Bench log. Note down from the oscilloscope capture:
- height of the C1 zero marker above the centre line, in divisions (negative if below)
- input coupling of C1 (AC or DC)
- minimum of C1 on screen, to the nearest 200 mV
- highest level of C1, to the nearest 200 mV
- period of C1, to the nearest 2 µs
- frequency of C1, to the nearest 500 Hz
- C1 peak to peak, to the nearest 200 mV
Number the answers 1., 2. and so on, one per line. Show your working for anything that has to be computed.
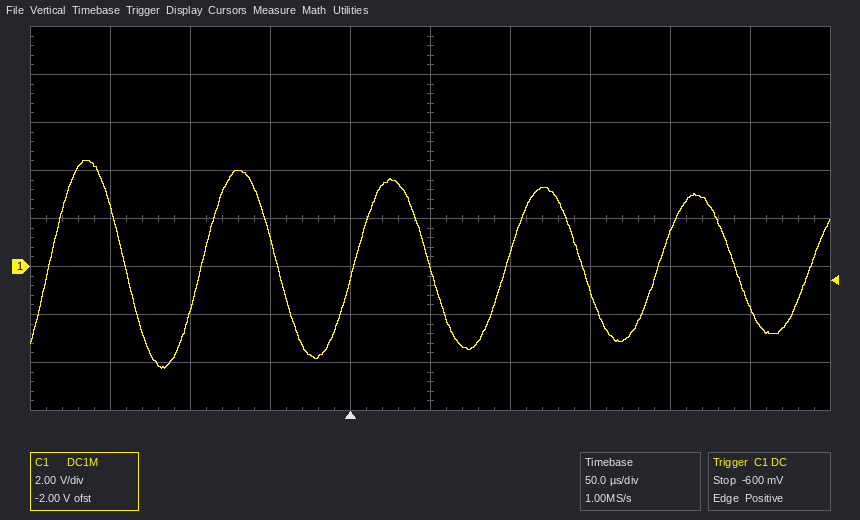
1. -1.0 div
2. DC
3. -4.2 V
4. 4.4 V
5. 96 µs
6. 1 / 96 µs ≈ 10.4 kHz, so 10.5 kHz to the nearest 500 Hz
7. 4.4 V − (-4.2 V) = 8.6 V
